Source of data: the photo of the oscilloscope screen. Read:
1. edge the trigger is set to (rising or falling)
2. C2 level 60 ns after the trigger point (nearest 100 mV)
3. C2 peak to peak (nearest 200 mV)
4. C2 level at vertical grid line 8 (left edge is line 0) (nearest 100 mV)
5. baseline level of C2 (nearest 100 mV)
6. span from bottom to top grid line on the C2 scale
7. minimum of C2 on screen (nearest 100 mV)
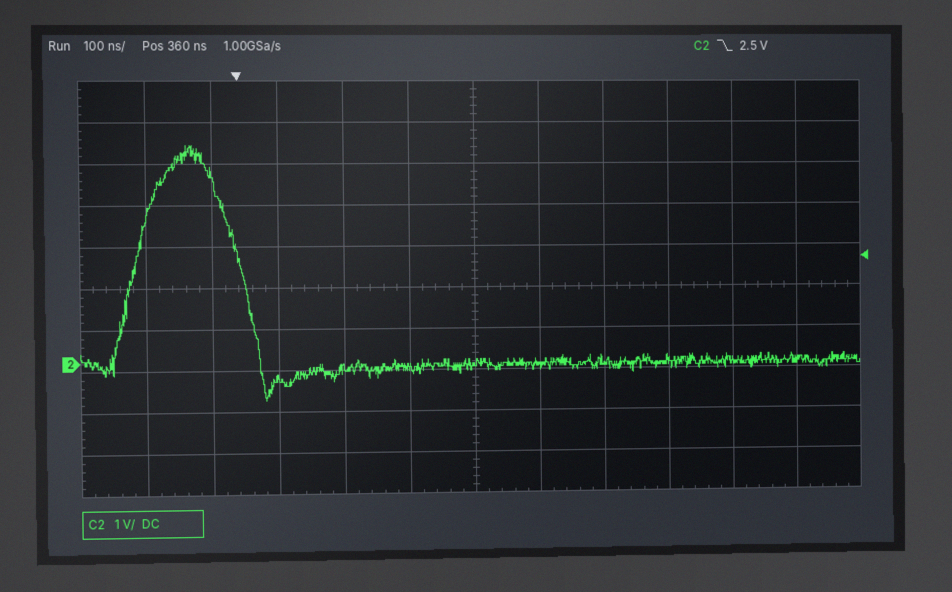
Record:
falling
-400 mV
6.2 V
0.0 V
-100 mV
10 V
-900 mV
